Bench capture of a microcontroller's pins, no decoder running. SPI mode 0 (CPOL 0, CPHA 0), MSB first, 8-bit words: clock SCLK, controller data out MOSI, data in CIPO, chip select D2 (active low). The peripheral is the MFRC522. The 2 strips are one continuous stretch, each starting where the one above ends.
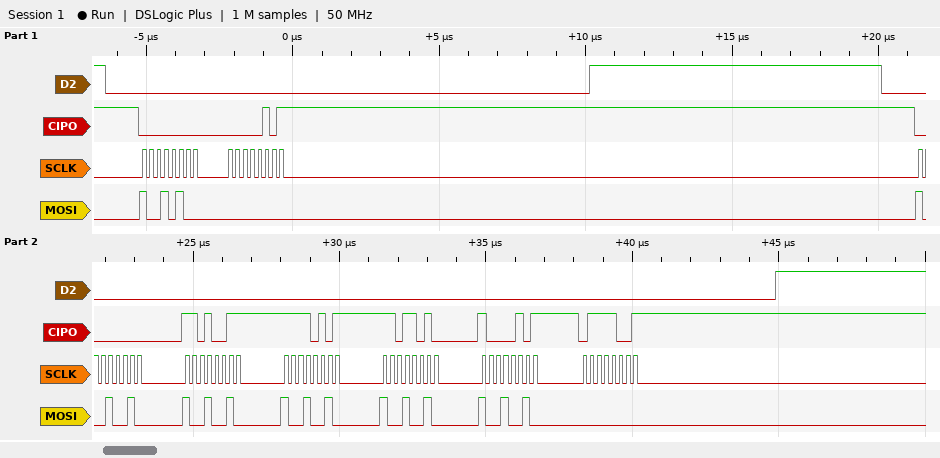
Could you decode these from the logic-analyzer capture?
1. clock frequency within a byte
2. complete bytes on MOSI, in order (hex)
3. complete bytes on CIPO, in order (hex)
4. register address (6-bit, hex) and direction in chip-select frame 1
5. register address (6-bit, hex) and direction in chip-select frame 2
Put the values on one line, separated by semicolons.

4 MHz; 94 00 92 92 92 92 92 00; 00 05 00 D3 F5 DA 85 79; 0x0A read; 0x09 read
